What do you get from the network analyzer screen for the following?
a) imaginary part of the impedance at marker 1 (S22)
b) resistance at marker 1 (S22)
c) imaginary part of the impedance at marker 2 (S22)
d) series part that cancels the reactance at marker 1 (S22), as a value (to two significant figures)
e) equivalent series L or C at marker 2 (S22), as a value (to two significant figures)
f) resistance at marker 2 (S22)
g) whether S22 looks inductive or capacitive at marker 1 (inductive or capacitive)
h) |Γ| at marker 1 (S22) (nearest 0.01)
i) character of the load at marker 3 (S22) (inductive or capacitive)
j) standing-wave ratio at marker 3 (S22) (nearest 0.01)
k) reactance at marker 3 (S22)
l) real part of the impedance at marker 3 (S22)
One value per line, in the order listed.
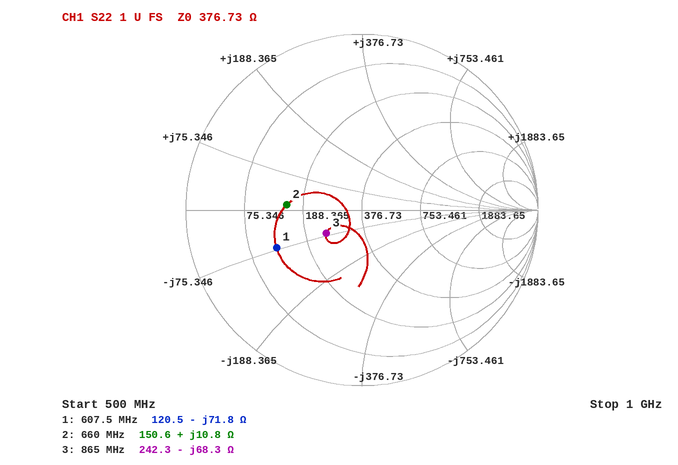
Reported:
-71.8 Ω
120.5 Ω
+10.8 Ω
19 nH
2.6 nH
150.6 Ω
capacitive
0.53
capacitive
1.64
-68.3 Ω
242.3 Ω
